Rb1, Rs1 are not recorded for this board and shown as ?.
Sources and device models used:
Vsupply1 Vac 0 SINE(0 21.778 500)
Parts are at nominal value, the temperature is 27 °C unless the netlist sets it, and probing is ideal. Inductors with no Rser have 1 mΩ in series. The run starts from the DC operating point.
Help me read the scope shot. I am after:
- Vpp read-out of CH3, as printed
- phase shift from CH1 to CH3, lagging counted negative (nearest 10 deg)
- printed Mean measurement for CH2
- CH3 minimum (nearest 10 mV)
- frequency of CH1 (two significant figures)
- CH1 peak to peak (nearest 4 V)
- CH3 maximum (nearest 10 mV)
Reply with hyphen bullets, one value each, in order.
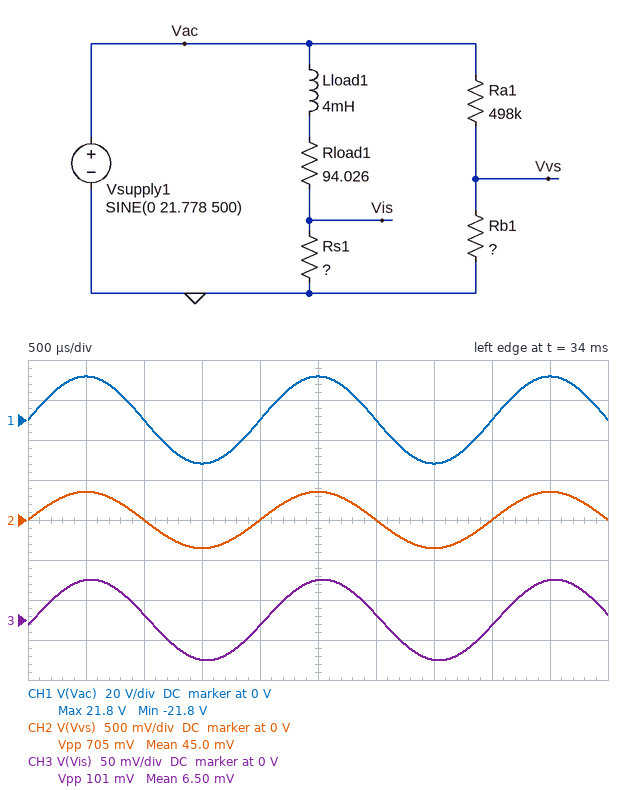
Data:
- 101 mV
- -10 deg
- 45.0 mV
- -50 mV
- 500 Hz
- 44 V
- 50 mV
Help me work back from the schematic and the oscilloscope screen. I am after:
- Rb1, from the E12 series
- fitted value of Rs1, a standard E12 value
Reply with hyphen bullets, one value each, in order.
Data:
- 8.2 kΩ
- 0.22 Ω
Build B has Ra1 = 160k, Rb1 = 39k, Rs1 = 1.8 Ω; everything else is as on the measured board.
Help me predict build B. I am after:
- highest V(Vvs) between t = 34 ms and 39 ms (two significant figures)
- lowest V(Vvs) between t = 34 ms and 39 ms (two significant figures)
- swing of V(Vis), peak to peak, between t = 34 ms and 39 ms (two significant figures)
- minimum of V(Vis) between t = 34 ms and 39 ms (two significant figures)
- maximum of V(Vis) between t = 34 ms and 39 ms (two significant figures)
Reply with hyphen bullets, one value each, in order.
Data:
- 4.3 V
- -4.3 V
- 810 mV
- -410 mV
- 410 mV
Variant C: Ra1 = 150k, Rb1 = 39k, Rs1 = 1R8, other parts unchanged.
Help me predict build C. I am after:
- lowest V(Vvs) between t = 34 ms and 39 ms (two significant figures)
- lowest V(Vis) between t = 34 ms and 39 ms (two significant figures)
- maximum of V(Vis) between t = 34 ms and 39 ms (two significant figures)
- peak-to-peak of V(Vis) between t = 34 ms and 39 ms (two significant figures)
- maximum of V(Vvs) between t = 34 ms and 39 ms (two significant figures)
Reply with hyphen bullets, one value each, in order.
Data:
- -4.5 V
- -410 mV
- 410 mV
- 810 mV
- 4.5 V
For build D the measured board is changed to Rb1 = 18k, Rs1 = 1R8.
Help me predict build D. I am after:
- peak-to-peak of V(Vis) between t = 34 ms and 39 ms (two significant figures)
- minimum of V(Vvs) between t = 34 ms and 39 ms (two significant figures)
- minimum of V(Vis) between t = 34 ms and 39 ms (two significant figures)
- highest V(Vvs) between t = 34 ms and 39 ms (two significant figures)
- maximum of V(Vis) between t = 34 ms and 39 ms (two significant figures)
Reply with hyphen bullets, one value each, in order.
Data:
- 810 mV
- -760 mV
- -410 mV
- 760 mV
- 410 mV
